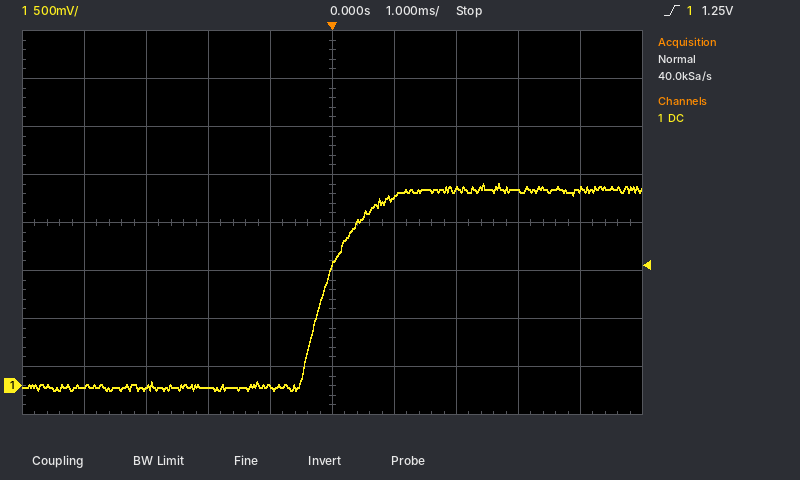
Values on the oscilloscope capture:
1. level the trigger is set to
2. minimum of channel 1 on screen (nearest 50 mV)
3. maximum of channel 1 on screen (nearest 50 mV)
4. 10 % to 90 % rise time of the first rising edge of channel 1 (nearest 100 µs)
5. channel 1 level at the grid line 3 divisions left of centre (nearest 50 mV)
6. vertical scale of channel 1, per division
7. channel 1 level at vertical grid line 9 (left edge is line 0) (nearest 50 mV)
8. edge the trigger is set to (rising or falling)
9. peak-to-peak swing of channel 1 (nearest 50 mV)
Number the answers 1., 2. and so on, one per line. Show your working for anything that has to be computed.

1. 1.25 V
2. -50 mV
3. 2.10 V
4. 1.1 ms
5. 0 mV
6. 500 mV
7. 2.05 V
8. rising
9. 2.10 V − (-50 mV) = 2.15 V
